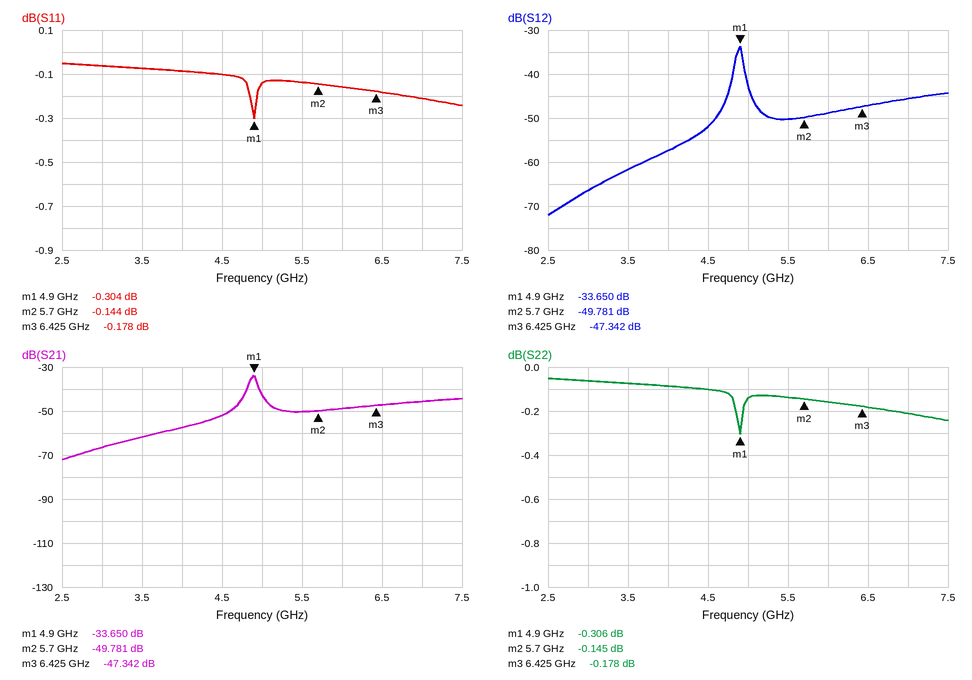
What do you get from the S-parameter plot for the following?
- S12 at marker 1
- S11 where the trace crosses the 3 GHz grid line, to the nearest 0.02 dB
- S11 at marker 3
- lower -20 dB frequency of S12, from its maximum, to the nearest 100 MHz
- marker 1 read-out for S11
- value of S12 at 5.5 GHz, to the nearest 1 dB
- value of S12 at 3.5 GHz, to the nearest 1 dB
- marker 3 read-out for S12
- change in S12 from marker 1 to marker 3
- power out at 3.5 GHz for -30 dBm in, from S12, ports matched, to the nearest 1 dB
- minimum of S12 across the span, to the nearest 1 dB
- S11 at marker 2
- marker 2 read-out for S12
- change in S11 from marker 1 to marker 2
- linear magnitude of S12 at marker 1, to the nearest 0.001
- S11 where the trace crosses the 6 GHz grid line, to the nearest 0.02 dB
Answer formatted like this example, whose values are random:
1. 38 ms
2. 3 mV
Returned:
1. -33.650 dB
2. -0.06 dB
3. -0.178 dB
4. 4.4 GHz
5. -0.304 dB
6. -50 dB
7. -62 dB
8. -47.342 dB
9. -13.692 dB
10. -92 dBm
11. -72 dB
12. -0.144 dB
13. -49.781 dB
14. 0.160 dB
15. 0.021
16. -0.16 dB
